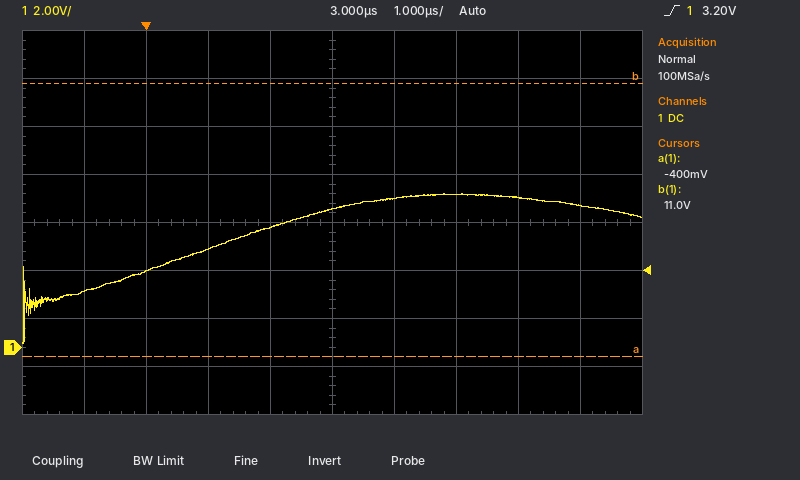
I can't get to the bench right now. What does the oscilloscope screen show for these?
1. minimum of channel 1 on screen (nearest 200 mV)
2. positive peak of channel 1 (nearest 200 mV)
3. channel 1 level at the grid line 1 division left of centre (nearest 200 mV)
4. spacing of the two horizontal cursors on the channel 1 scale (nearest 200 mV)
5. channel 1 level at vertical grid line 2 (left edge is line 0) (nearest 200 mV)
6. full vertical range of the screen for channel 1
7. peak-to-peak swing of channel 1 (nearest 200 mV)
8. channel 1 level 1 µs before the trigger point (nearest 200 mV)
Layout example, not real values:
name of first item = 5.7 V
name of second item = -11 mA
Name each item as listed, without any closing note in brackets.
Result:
minimum of channel 1 on screen = 200 mV
positive peak of channel 1 = 6.4 V
channel 1 level at the grid line 1 division left of centre = 5.0 V
spacing of the two horizontal cursors on the channel 1 scale = 11.4 V
channel 1 level at vertical grid line 2 (left edge is line 0) = 3.2 V
full vertical range of the screen for channel 1 = 16 V
peak-to-peak swing of channel 1 = 6.2 V
channel 1 level 1 µs before the trigger point = 2.4 V
